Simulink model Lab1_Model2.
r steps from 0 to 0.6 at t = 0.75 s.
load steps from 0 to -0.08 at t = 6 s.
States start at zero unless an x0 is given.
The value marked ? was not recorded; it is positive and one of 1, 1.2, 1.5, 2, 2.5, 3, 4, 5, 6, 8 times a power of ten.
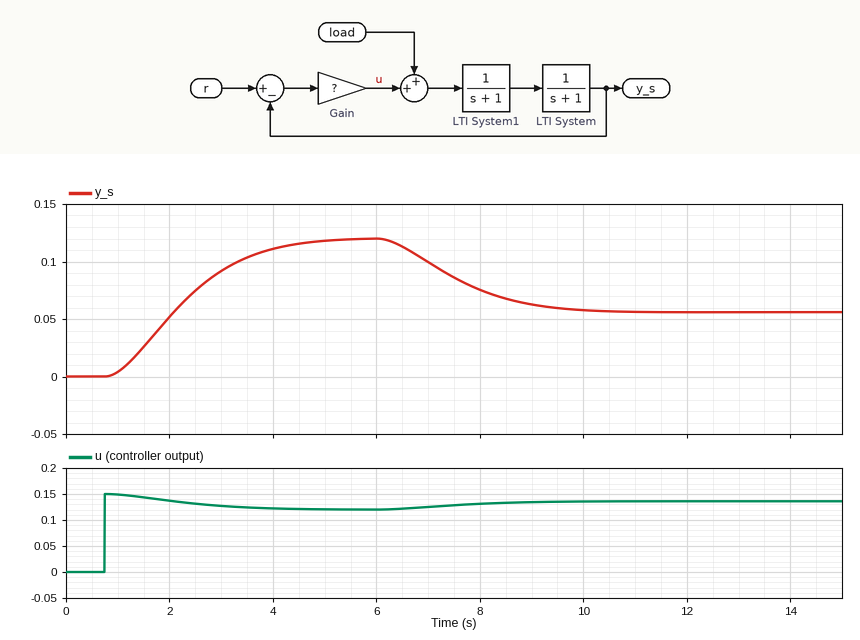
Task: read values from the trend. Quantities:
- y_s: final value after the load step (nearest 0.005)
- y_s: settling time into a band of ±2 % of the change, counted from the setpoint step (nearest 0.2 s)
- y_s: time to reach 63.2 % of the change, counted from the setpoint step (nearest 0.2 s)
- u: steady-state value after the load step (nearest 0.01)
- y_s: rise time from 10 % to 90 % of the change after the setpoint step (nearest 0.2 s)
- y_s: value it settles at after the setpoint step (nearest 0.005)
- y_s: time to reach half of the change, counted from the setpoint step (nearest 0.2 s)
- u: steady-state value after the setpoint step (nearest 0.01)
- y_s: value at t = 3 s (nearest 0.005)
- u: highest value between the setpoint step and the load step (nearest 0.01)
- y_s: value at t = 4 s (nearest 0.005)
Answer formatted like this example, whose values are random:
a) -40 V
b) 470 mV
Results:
a) 0.055
b) 4.2 s
c) 1.8 s
d) 0.14
e) 2.6 s
f) 0.120
g) 1.4 s
h) 0.12
i) 0.090
j) 0.15
k) 0.110
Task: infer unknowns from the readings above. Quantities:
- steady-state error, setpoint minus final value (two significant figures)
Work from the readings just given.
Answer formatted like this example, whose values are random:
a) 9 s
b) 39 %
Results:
a) 0.48
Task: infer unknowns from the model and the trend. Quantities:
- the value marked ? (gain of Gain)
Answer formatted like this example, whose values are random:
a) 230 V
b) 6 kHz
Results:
a) 0.25
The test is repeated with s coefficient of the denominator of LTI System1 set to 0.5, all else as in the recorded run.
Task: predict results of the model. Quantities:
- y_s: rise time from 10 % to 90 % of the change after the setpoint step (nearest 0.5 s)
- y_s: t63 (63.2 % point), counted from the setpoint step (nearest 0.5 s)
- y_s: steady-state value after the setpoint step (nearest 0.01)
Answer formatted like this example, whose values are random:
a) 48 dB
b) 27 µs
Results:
a) 2.0 s
b) 1.5 s
c) 0.12
